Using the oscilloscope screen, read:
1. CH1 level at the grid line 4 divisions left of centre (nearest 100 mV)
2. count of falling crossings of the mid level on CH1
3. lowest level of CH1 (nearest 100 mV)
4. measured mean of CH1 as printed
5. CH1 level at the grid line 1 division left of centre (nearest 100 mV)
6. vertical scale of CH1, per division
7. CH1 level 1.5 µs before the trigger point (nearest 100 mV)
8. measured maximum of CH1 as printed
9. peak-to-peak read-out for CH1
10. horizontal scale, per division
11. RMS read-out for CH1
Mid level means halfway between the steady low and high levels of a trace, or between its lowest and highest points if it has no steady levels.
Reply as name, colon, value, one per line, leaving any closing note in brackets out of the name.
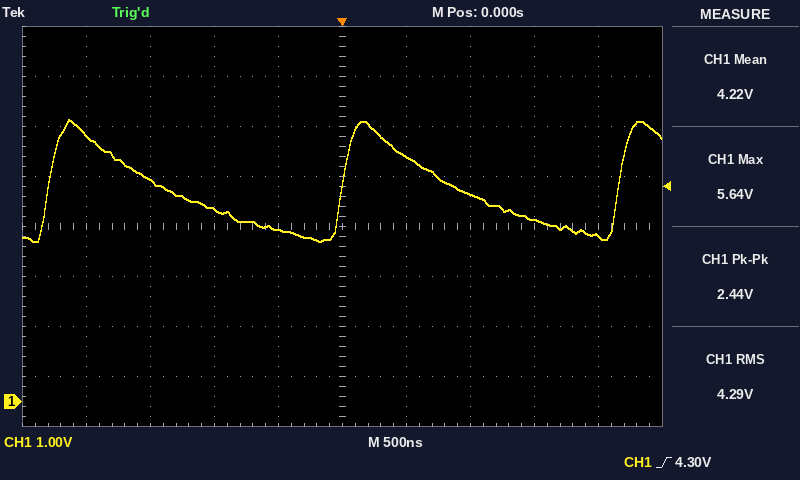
CH1 level at the grid line 4 divisions left of centre: 5.3 V
count of falling crossings of the mid level on CH1: 2
lowest level of CH1: 3.2 V
measured mean of CH1 as printed: 4.22 V
CH1 level at the grid line 1 division left of centre: 3.4 V
vertical scale of CH1, per division: 1 V
CH1 level 1.5 µs before the trigger point: 4.4 V
measured maximum of CH1 as printed: 5.64 V
peak-to-peak read-out for CH1: 2.44 V
horizontal scale, per division: 500 ns
RMS read-out for CH1: 4.29 V
